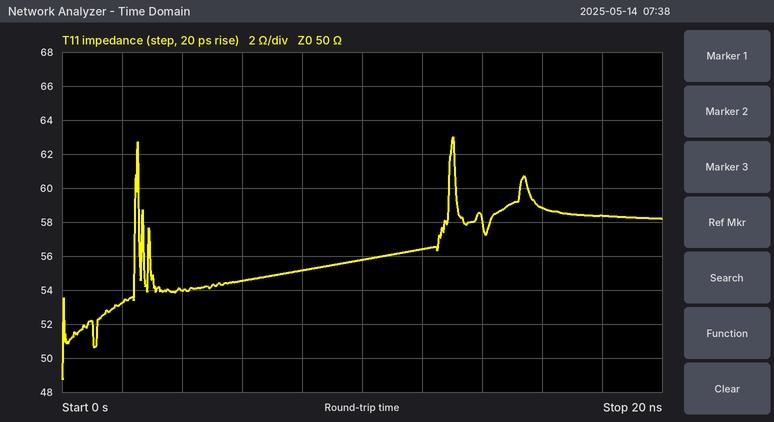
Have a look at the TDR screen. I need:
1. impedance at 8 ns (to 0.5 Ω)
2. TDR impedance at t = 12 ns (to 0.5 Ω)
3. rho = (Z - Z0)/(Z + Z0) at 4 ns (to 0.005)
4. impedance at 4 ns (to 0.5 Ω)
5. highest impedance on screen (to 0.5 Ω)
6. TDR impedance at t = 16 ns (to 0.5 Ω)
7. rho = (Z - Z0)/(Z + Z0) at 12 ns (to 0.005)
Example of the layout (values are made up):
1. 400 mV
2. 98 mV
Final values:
1. 55.0 Ω
2. 56.5 Ω
3. +0.040
4. 54.0 Ω
5. 63.0 Ω
6. 59.0 Ω
7. +0.060
